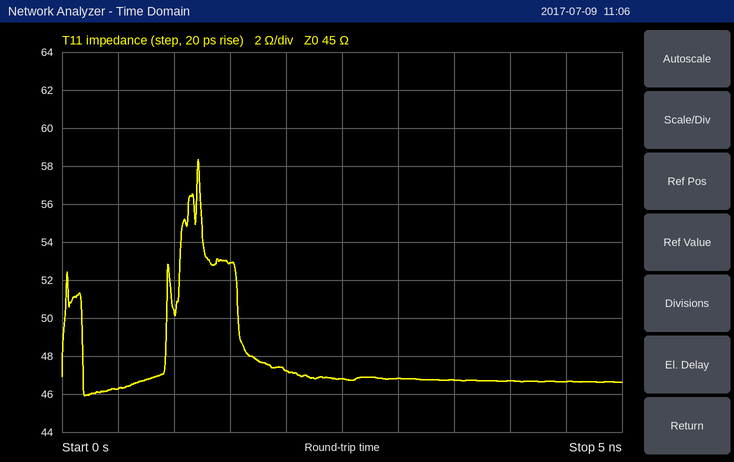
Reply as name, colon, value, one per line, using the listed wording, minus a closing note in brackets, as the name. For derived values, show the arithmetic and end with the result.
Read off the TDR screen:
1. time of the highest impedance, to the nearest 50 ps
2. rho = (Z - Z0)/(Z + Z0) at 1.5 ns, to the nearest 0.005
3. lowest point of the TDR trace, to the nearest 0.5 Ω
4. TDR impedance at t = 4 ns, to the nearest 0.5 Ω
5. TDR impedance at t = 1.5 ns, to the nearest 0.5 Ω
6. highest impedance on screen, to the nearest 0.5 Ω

time of the highest impedance, to the nearest 50 ps: 1.20 ns
rho = (Z - Z0)/(Z + Z0) at 1.5 ns, to the nearest 0.005: (53 − 45)/(53 + 45) ≈ +0.0816, so +0.080 to the nearest 0.005
lowest point of the TDR trace, to the nearest 0.5 Ω: 46.0 Ω
TDR impedance at t = 4 ns, to the nearest 0.5 Ω: 46.5 Ω
TDR impedance at t = 1.5 ns, to the nearest 0.5 Ω: 53.0 Ω
highest impedance on screen, to the nearest 0.5 Ω: 58.5 Ω
